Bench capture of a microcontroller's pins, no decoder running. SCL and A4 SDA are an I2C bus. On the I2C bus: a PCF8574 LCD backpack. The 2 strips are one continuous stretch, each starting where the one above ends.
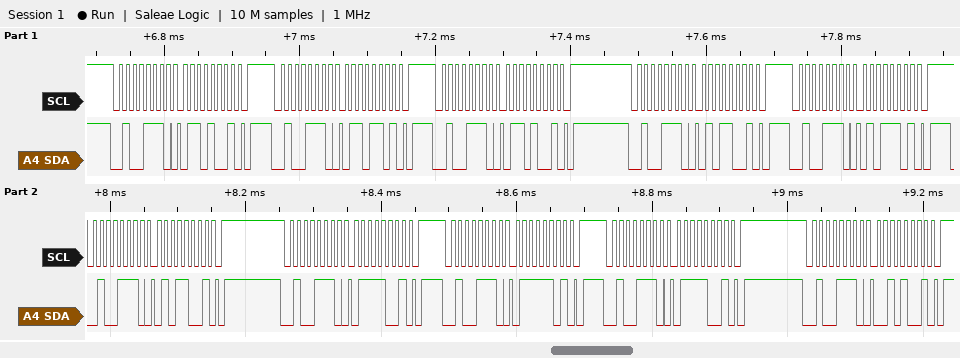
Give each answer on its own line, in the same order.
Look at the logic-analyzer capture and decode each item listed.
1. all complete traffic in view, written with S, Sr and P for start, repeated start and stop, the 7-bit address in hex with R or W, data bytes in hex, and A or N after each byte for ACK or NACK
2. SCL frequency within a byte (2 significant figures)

S 27W A 69 A P S 27W A 6D A P S 27W A 69 A P S 27W A 59 A P S 27W A 5D A P S 27W A 59 A P S 27W A 79 A P S 27W A 7D A P S 27W A 79 A P S 27W A 29 A P
100 kHz
